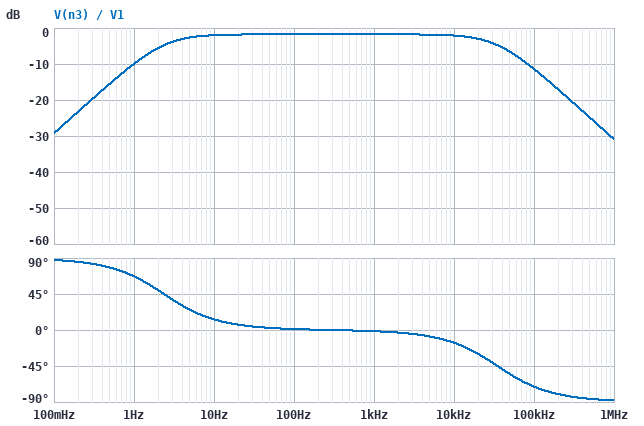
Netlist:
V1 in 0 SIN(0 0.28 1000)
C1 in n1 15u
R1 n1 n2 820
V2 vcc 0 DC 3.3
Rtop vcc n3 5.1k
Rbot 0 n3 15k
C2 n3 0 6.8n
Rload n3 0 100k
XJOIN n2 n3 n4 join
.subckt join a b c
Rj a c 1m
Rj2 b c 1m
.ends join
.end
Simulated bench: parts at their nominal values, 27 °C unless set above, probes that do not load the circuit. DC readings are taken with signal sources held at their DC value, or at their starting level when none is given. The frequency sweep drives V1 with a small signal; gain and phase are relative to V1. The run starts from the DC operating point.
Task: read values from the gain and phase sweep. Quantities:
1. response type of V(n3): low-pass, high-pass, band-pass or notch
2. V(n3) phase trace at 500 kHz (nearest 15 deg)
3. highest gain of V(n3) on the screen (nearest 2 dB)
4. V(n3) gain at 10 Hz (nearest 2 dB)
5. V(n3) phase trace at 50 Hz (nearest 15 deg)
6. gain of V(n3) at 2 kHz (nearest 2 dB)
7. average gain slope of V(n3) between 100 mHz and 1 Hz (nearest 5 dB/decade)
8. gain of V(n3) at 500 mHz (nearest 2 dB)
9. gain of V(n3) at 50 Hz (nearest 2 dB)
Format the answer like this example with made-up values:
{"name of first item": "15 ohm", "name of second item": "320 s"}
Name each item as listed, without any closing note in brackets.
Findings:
{"response type of V(n3): low-pass, high-pass, band-pass or notch": "band-pass", "V(n3) phase trace at 500 kHz": "-90 deg", "highest gain of V(n3) on the screen": "-2 dB", "V(n3) gain at 10 Hz": "-2 dB", "V(n3) phase trace at 50 Hz": "0 deg", "gain of V(n3) at 2 kHz": "-2 dB", "average gain slope of V(n3) between 100 mHz and 1 Hz": "20 dB/decade", "gain of V(n3) at 500 mHz": "-16 dB", "gain of V(n3) at 50 Hz": "-2 dB"}
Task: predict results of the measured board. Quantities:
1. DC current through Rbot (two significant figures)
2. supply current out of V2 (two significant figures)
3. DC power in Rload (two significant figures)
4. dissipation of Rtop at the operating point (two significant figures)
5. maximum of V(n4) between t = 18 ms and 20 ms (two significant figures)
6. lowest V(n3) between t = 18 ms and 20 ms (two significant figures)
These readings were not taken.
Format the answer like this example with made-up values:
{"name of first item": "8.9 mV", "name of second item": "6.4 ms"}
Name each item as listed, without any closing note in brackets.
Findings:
{"DC current through Rbot": "160 µA", "supply current out of V2": "180 µA", "DC power in Rload": "56 µW", "dissipation of Rtop at the operating point": "170 µW", "maximum of V(n4) between t = 18 ms and 20 ms": "2.6 V", "lowest V(n3) between t = 18 ms and 20 ms": "2.1 V"}
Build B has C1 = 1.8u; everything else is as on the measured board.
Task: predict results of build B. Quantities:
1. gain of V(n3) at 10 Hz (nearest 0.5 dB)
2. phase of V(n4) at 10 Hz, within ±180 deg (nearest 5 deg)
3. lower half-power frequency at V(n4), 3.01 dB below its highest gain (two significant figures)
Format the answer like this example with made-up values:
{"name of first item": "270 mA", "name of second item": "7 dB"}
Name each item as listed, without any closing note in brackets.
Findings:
{"gain of V(n3) at 10 Hz": "-8.5 dB", "phase of V(n4) at 10 Hz, within ±180 deg": "65 deg", "lower half-power frequency at V(n4), 3.01 dB below its highest gain": "20 Hz"}
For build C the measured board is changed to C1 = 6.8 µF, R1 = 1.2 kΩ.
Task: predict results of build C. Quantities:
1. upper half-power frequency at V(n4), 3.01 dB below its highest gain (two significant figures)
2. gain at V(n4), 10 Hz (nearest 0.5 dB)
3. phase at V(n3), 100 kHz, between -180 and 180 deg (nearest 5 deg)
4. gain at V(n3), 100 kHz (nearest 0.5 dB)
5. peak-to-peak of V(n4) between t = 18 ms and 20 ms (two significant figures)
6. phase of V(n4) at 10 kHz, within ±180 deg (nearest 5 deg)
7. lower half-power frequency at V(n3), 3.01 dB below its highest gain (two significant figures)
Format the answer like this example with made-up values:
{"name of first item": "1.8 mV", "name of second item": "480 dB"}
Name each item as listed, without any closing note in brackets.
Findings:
{"upper half-power frequency at V(n4), 3.01 dB below its highest gain": "26 kHz", "gain at V(n4), 10 Hz": "-3.5 dB", "phase at V(n3), 100 kHz, between -180 and 180 deg": "-75 deg", "gain at V(n3), 100 kHz": "-14.5 dB", "peak-to-peak of V(n4) between t = 18 ms and 20 ms": "420 mV", "phase of V(n4) at 10 kHz, within ±180 deg": "-20 deg", "lower half-power frequency at V(n3), 3.01 dB below its highest gain": "4.8 Hz"}
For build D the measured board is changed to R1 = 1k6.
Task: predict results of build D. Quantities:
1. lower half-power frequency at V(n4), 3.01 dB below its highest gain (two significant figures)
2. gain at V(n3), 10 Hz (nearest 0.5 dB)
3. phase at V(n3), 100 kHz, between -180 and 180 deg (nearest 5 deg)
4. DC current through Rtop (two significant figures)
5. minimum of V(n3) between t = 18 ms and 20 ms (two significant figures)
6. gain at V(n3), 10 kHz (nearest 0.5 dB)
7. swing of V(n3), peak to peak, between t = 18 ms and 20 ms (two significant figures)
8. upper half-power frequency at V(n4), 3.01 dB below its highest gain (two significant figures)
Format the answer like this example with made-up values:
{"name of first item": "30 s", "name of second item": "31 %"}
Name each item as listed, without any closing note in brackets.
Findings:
{"lower half-power frequency at V(n4), 3.01 dB below its highest gain": "2.0 Hz", "gain at V(n3), 10 Hz": "-3.5 dB", "phase at V(n3), 100 kHz, between -180 and 180 deg": "-80 deg", "DC current through Rtop": "180 µA", "minimum of V(n3) between t = 18 ms and 20 ms": "2.2 V", "gain at V(n3), 10 kHz": "-4.0 dB", "swing of V(n3), peak to peak, between t = 18 ms and 20 ms": "390 mV", "upper half-power frequency at V(n4), 3.01 dB below its highest gain": "21 kHz"}
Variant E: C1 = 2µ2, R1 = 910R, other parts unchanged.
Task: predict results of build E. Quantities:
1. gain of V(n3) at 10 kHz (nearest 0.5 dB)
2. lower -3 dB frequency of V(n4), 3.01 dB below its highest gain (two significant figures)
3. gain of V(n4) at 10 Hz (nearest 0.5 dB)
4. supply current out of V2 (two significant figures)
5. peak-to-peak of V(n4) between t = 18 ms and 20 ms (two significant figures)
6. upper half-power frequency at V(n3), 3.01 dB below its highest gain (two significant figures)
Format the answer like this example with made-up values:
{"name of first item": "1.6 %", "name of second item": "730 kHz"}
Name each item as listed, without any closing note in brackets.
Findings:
{"gain of V(n3) at 10 kHz": "-2.5 dB", "lower -3 dB frequency of V(n4), 3.01 dB below its highest gain": "16 Hz", "gain of V(n4) at 10 Hz": "-7.5 dB", "supply current out of V2": "180 µA", "peak-to-peak of V(n4) between t = 18 ms and 20 ms": "450 mV", "upper half-power frequency at V(n3), 3.01 dB below its highest gain": "32 kHz"}
